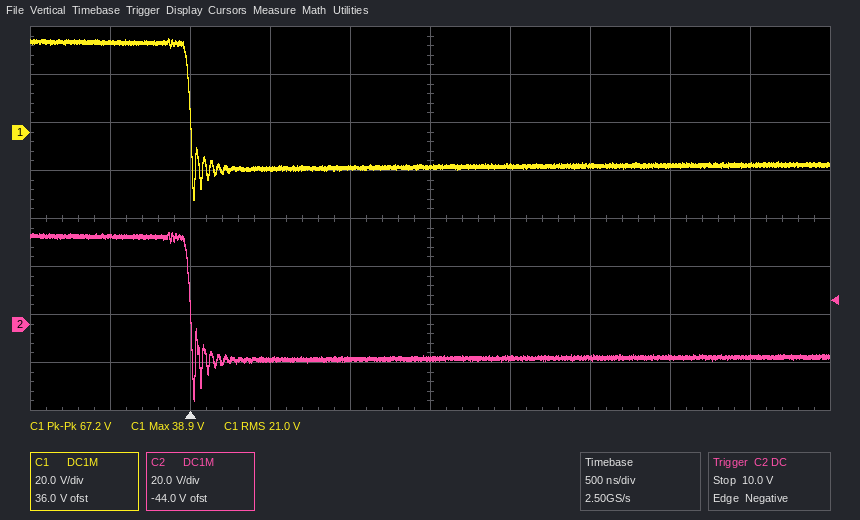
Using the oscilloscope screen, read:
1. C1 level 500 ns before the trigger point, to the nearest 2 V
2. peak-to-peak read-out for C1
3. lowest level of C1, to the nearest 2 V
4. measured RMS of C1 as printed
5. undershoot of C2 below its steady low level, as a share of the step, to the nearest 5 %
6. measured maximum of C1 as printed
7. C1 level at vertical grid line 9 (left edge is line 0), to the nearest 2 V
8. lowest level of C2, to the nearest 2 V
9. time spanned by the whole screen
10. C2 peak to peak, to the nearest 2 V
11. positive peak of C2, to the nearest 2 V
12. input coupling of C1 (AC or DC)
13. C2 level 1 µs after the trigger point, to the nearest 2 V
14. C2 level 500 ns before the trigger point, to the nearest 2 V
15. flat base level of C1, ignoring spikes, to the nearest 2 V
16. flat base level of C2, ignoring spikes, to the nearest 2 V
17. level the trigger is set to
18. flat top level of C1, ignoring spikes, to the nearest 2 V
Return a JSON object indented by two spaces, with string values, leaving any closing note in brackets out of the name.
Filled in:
{
  "C1 level 500 ns before the trigger point, to the nearest 2 V": "38 V",
  "peak-to-peak read-out for C1": "67.2 V",
  "lowest level of C1, to the nearest 2 V": "-28 V",
  "measured RMS of C1 as printed": "21.0 V",
  "undershoot of C2 below its steady low level, as a share of the step, to the nearest 5 %": "35 %",
  "measured maximum of C1 as printed": "38.9 V",
  "C1 level at vertical grid line 9 (left edge is line 0), to the nearest 2 V": "-14 V",
  "lowest level of C2, to the nearest 2 V": "-32 V",
  "time spanned by the whole screen": "5 µs",
  "C2 peak to peak, to the nearest 2 V": "70 V",
  "positive peak of C2, to the nearest 2 V": "38 V",
  "input coupling of C1": "DC",
  "C2 level 1 µs after the trigger point, to the nearest 2 V": "-14 V",
  "C2 level 500 ns before the trigger point, to the nearest 2 V": "36 V",
  "flat base level of C1, ignoring spikes, to the nearest 2 V": "-14 V",
  "flat base level of C2, ignoring spikes, to the nearest 2 V": "-14 V",
  "level the trigger is set to": "10.0 V",
  "flat top level of C1, ignoring spikes, to the nearest 2 V": "38 V"
}
